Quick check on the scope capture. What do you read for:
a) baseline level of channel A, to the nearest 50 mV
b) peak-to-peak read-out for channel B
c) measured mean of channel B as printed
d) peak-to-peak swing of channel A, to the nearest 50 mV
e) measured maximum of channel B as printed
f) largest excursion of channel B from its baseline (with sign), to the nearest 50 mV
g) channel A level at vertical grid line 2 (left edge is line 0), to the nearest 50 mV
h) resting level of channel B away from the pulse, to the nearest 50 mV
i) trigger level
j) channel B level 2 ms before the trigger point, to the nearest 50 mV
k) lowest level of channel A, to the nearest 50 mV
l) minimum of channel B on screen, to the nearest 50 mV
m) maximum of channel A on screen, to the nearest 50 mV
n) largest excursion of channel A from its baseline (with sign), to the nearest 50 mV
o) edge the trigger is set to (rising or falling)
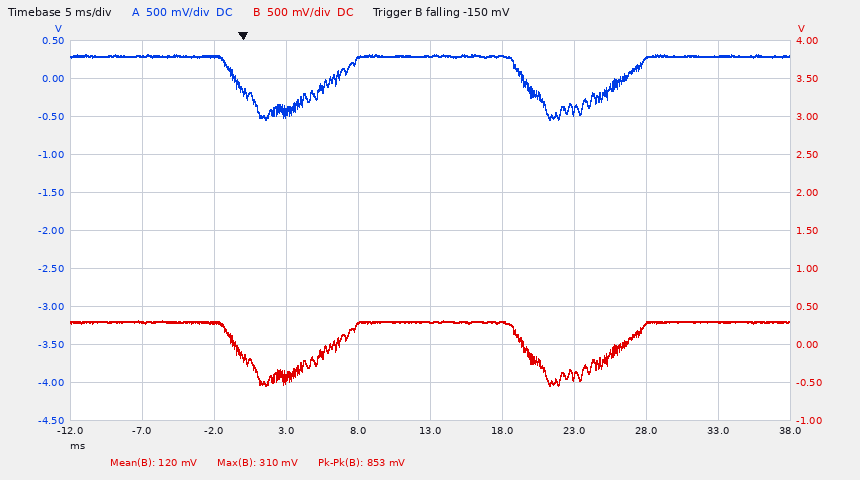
300 mV
853 mV
120 mV
850 mV
310 mV
-850 mV
300 mV
300 mV
-150 mV
300 mV
-550 mV
-550 mV
300 mV
-850 mV
falling
